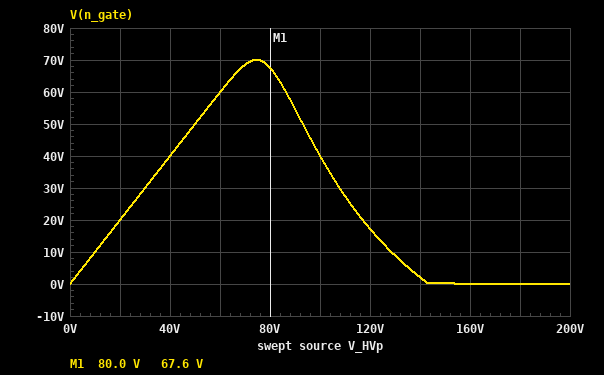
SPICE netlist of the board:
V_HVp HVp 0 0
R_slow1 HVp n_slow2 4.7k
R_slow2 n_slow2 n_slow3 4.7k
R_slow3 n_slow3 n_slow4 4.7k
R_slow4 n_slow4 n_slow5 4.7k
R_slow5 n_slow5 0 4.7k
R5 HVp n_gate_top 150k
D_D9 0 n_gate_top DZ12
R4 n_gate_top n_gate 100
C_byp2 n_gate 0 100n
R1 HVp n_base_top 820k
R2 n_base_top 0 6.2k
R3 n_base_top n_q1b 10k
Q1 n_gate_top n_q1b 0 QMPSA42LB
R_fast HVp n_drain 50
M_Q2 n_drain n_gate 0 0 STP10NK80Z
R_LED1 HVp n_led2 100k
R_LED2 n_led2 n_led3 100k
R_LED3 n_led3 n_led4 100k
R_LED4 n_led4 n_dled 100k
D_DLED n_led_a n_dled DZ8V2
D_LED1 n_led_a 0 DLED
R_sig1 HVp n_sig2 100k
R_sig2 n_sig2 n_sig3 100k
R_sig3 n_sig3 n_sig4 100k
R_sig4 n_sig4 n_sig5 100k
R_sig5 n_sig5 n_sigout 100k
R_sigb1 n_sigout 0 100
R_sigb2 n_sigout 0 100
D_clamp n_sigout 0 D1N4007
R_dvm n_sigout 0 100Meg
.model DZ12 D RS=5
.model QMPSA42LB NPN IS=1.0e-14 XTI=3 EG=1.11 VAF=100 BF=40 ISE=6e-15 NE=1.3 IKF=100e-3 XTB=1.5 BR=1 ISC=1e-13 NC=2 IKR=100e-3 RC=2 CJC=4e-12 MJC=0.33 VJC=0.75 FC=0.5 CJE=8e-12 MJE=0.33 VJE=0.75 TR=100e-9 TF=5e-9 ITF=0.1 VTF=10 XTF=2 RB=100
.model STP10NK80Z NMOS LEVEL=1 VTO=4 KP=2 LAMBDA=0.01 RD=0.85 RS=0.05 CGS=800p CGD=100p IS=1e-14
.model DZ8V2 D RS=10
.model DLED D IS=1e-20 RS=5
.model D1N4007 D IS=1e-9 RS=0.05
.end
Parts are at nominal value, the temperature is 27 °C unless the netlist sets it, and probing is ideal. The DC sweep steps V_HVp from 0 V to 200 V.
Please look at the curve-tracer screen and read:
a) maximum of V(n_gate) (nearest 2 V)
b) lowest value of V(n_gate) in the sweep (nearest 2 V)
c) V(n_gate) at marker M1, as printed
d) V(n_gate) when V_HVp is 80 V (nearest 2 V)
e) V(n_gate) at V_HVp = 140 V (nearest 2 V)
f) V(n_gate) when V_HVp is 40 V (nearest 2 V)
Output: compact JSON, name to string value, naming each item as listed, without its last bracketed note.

{"maximum of V(n_gate)": "70 V", "lowest value of V(n_gate) in the sweep": "0 V", "V(n_gate) at marker M1, as printed": "67.6 V", "V(n_gate) when V_HVp is 80 V": "68 V", "V(n_gate) at V_HVp = 140 V": "2 V", "V(n_gate) when V_HVp is 40 V": "40 V"}
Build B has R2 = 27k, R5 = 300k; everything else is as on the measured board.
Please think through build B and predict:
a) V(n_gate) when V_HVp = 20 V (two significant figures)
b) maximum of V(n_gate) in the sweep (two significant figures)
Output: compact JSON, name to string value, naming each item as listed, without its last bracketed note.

{"V(n_gate) when V_HVp = 20 V": "2.9 V", "maximum of V(n_gate) in the sweep": "15 V"}
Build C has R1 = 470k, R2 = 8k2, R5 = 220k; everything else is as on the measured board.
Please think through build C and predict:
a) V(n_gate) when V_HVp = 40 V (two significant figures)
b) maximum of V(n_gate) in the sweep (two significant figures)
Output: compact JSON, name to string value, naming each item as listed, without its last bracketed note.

{"V(n_gate) when V_HVp = 40 V": "4.3 V", "maximum of V(n_gate) in the sweep": "29 V"}
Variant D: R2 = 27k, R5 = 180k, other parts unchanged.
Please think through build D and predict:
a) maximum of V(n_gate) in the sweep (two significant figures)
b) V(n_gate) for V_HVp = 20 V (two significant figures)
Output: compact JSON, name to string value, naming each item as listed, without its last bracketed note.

{"maximum of V(n_gate) in the sweep": "15 V", "V(n_gate) for V_HVp = 20 V": "9.1 V"}
